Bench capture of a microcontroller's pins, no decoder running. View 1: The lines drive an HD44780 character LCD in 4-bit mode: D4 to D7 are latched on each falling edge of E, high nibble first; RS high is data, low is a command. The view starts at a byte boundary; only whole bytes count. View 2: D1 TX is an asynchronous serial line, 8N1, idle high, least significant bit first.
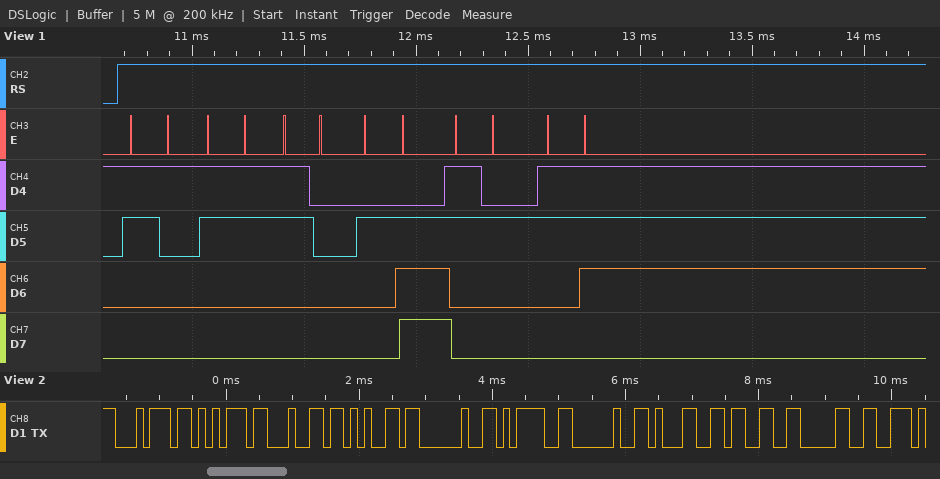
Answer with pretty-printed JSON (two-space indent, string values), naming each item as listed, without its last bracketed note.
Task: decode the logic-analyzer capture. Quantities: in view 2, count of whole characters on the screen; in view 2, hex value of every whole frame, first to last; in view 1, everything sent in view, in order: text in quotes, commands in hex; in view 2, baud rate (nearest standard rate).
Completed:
{
  "in view 2, count of whole characters on the screen": "10",
  "in view 2, hex value of every whole frame, first to last": "74 75 64 65 20 3D 20 31 33 30",
  "in view 1, everything sent in view, in order: text in quotes, commands in hex": "\"130.27\"",
  "in view 2, baud rate": "9600 baud"
}
